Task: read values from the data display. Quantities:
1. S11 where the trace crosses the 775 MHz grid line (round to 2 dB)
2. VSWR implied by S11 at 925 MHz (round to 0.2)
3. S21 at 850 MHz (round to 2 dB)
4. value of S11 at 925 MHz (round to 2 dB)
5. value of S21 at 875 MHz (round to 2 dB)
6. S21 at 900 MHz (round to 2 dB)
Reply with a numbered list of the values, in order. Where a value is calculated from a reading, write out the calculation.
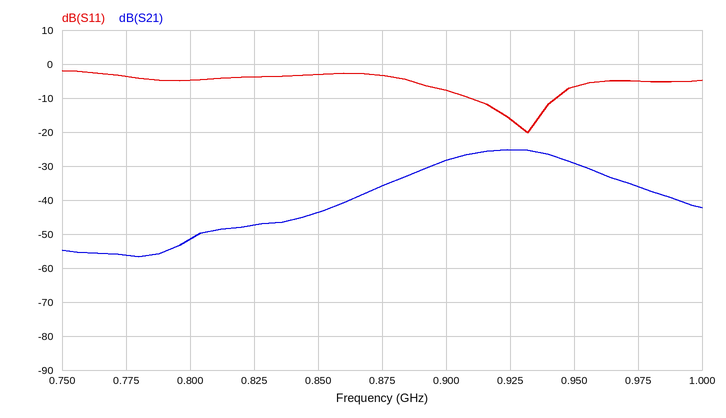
1. -4 dB
2. |Γ| = 10^(-16/20) = 0.1585; VSWR = (1 + 0.1585)/(1 − 0.1585) ≈ 1.4
3. -44 dB
4. -16 dB
5. -36 dB
6. -28 dB
